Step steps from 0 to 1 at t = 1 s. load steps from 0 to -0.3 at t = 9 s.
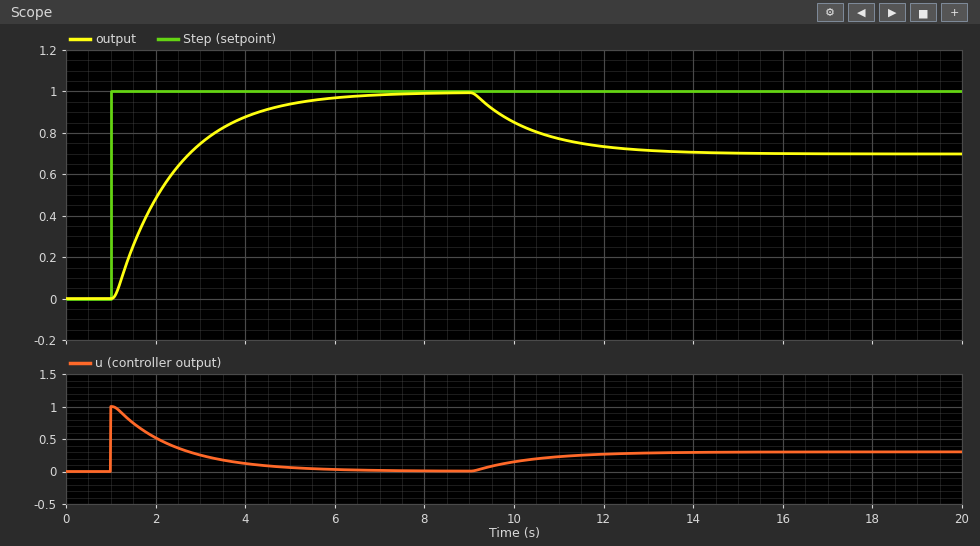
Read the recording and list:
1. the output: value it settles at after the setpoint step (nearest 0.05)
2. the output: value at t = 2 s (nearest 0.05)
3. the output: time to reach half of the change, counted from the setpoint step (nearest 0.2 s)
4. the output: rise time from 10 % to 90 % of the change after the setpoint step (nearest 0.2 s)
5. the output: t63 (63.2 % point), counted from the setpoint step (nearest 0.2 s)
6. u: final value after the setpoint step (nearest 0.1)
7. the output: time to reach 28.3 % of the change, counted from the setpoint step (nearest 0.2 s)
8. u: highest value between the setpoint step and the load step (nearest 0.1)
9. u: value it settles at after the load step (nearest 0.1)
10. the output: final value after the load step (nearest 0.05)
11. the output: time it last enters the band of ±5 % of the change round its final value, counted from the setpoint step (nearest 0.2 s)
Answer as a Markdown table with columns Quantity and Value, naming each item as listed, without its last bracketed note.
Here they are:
| Quantity | Value |
|---|---|
| the output: value it settles at after the setpoint step | 1.00 |
| the output: value at t = 2 s | 0.50 |
| the output: time to reach half of the change, counted from the setpoint step | 1.0 s |
| the output: rise time from 10 % to 90 % of the change after the setpoint step | 3.0 s |
| the output: t63 (63.2 % point), counted from the setpoint step | 1.4 s |
| u: final value after the setpoint step | 0.0 |
| the output: time to reach 28.3 % of the change, counted from the setpoint step | 0.6 s |
| u: highest value between the setpoint step and the load step | 1.0 |
| u: value it settles at after the load step | 0.3 |
| the output: final value after the load step | 0.70 |
| the output: time it last enters the band of ±5 % of the change round its final value, counted from the setpoint step | 4.2 s |
